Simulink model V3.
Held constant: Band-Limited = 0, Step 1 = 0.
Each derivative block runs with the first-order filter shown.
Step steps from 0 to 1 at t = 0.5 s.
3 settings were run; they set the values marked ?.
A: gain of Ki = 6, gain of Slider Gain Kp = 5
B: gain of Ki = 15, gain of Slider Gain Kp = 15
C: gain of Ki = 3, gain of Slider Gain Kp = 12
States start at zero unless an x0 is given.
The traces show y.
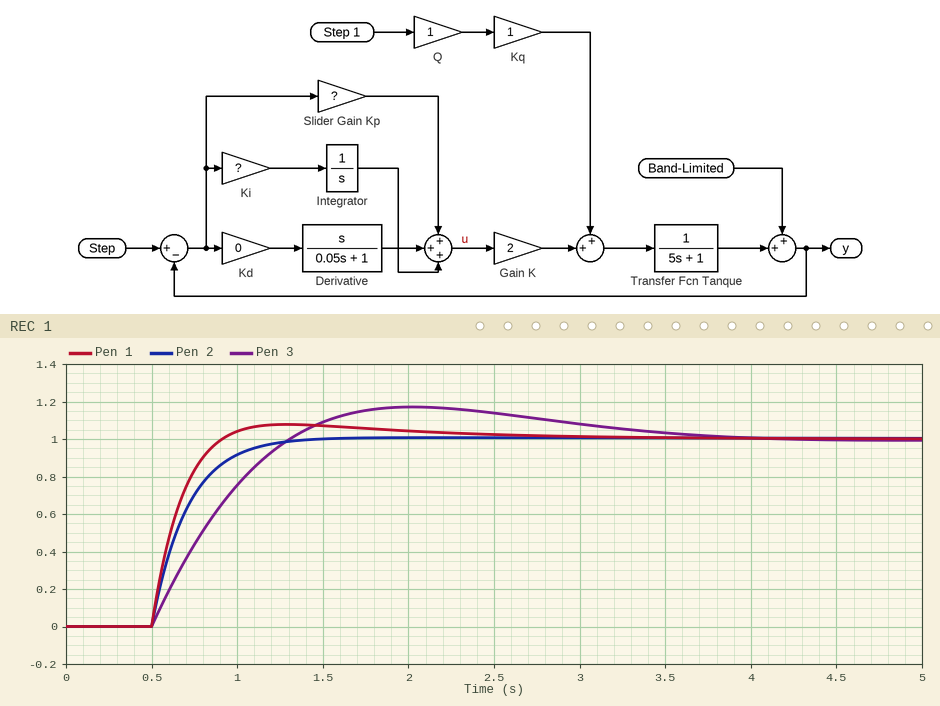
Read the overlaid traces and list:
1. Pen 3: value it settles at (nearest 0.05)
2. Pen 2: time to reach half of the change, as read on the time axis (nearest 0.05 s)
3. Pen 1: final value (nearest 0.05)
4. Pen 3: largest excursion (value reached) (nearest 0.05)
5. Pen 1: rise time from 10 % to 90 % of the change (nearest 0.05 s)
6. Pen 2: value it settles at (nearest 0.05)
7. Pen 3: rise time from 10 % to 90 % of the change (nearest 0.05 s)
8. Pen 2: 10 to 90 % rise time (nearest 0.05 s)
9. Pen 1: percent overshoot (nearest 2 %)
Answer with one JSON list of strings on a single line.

["1.00", "0.65 s", "1.00", "1.15", "0.30 s", "1.00", "0.60 s", "0.45 s", "8 %"]
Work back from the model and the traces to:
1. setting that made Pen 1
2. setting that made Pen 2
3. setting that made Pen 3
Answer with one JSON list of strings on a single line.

["B", "C", "A"]
